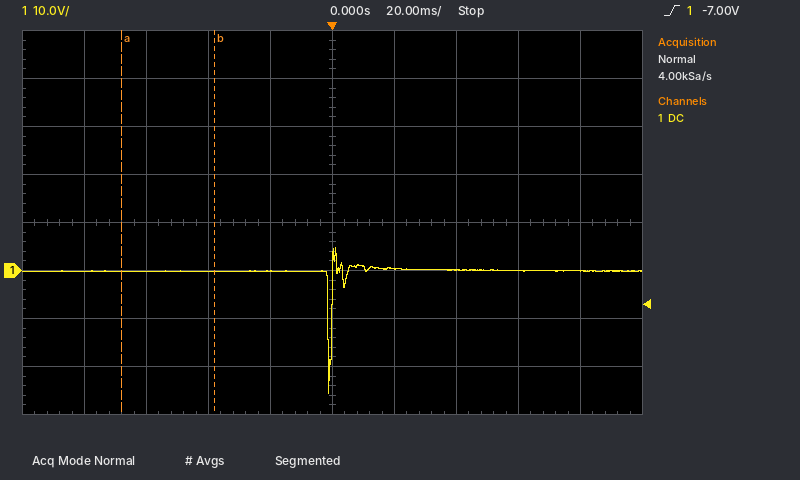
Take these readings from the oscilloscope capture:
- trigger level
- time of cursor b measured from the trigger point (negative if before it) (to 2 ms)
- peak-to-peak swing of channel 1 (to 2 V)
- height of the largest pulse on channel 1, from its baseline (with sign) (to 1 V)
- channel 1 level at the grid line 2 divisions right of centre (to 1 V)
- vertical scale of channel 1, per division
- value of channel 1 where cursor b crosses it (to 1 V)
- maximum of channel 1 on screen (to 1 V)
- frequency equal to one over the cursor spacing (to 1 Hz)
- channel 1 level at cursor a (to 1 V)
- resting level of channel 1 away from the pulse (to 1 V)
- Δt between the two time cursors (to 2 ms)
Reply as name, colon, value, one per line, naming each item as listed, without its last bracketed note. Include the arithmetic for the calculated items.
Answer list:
trigger level: -7.00 V
time of cursor b measured from the trigger point (negative if before it): -38 ms
peak-to-peak swing of channel 1: 30 V
height of the largest pulse on channel 1, from its baseline (with sign): -25 V
channel 1 level at the grid line 2 divisions right of centre: 0 V
vertical scale of channel 1, per division: 10 V
value of channel 1 where cursor b crosses it: 0 V
maximum of channel 1 on screen: 5 V
frequency equal to one over the cursor spacing: 1 / 30 ms ≈ 33 Hz
channel 1 level at cursor a: 0 V
resting level of channel 1 away from the pulse: 0 V
Δt between the two time cursors: 30 ms
